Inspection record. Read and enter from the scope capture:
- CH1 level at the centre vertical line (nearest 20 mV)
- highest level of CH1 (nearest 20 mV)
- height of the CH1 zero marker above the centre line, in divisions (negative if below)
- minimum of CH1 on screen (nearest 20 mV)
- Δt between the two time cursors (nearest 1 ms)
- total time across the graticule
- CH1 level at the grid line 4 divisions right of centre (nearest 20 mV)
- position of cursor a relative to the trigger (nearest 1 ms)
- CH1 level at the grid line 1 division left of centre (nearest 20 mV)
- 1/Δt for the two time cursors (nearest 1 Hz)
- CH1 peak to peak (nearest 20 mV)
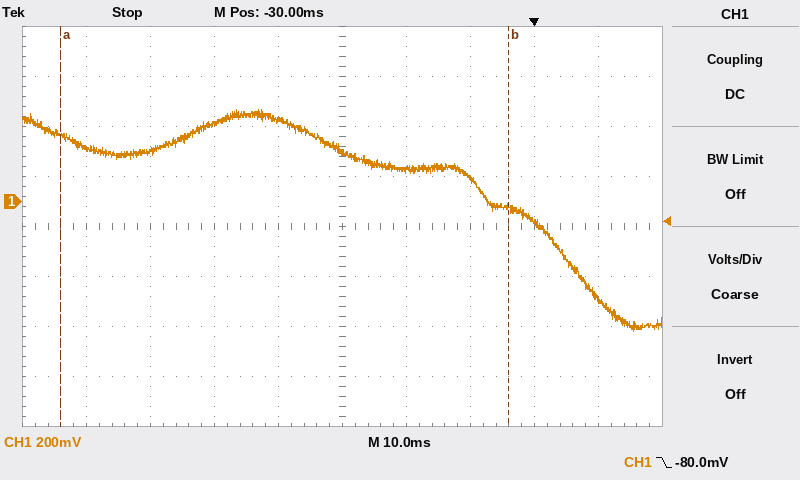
200 mV
360 mV
+0.5 div
-520 mV
70 ms
100 ms
-380 mV
-74 ms
320 mV
14 Hz
880 mV
